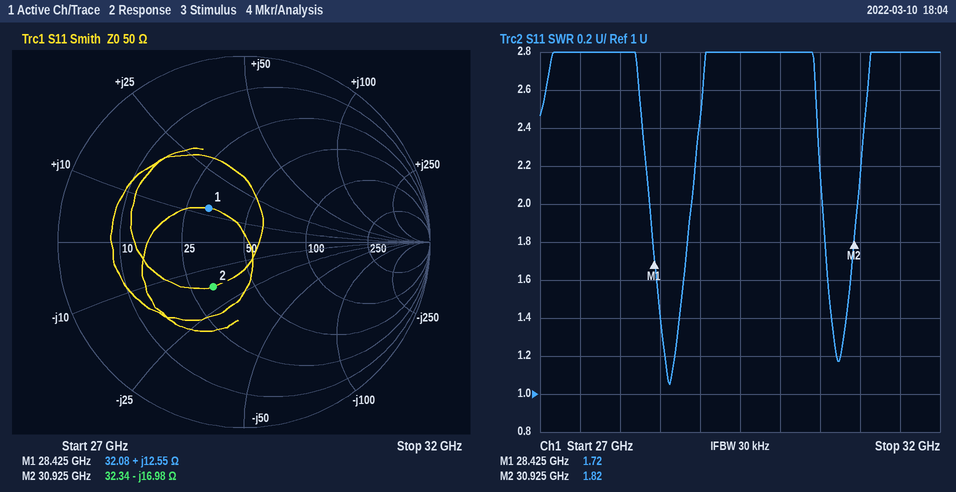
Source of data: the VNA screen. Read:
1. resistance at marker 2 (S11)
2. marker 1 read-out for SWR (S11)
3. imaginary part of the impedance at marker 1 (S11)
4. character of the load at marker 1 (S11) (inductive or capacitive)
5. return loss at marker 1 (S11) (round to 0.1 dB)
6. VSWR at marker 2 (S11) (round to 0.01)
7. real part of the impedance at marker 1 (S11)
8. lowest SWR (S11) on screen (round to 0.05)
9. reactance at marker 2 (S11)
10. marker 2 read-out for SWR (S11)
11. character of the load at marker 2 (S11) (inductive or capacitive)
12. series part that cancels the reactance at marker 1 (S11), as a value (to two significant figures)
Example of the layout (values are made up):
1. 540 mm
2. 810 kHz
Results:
1. 32.34 Ω
2. 1.72
3. +12.55 Ω
4. inductive
5. 11.6 dB
6. 1.82
7. 32.08 Ω
8. 1.05
9. -16.98 Ω
10. 1.82
11. capacitive
12. 450 fF
